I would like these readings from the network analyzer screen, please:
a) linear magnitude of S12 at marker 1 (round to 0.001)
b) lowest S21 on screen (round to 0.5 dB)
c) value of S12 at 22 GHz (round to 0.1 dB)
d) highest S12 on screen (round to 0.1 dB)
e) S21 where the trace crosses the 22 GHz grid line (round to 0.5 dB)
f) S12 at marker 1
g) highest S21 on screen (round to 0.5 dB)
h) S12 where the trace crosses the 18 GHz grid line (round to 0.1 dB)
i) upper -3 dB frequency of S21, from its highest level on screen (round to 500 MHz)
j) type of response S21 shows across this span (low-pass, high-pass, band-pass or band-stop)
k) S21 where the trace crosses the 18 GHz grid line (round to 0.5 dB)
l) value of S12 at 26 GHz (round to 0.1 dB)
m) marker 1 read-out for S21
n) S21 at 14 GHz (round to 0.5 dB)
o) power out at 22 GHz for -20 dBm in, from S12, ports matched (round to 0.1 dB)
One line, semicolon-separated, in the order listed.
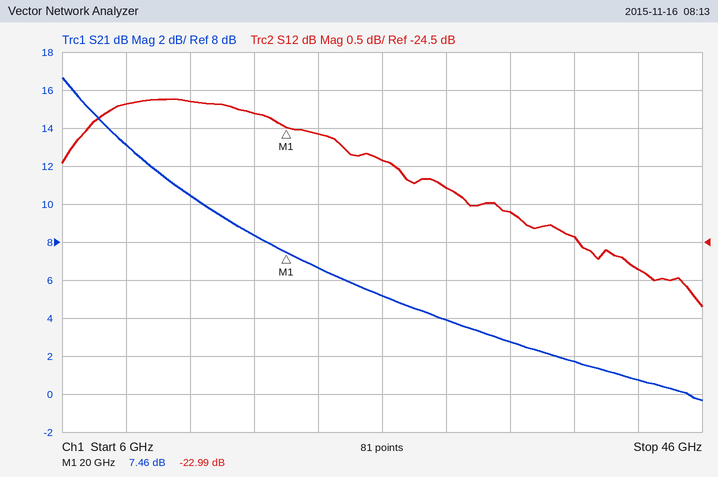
0.071; -0.5 dB; -23.1 dB; -22.6 dB; 6.5 dB; -22.99 dB; 16.5 dB; -22.8 dB; 9.5 GHz; low-pass; 8.5 dB; -23.4 dB; 7.46 dB; 10.5 dB; -43.1 dBm
